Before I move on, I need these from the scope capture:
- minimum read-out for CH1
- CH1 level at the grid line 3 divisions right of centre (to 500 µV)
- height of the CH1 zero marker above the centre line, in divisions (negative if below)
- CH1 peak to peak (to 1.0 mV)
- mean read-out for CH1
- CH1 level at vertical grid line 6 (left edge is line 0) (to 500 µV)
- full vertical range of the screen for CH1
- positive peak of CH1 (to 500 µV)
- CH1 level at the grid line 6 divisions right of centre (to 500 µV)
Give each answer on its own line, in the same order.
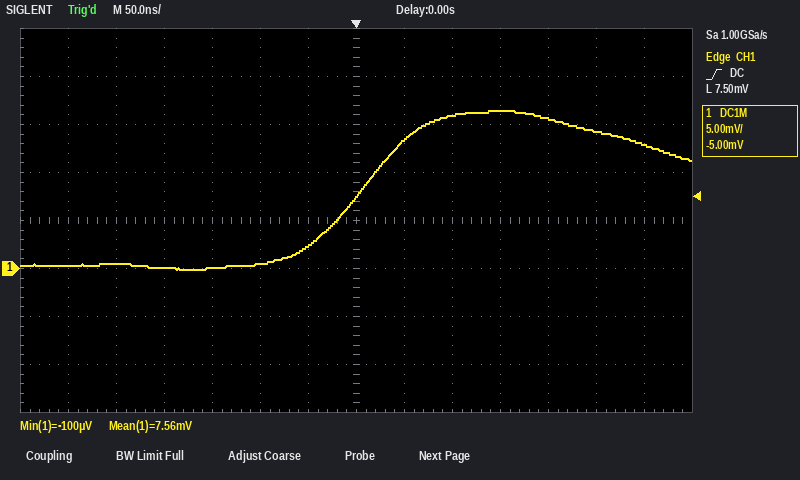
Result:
-100 µV
16.5 mV
-1.0 div
17.0 mV
7.56 mV
2.5 mV
40 mV
16.5 mV
13.0 mV
